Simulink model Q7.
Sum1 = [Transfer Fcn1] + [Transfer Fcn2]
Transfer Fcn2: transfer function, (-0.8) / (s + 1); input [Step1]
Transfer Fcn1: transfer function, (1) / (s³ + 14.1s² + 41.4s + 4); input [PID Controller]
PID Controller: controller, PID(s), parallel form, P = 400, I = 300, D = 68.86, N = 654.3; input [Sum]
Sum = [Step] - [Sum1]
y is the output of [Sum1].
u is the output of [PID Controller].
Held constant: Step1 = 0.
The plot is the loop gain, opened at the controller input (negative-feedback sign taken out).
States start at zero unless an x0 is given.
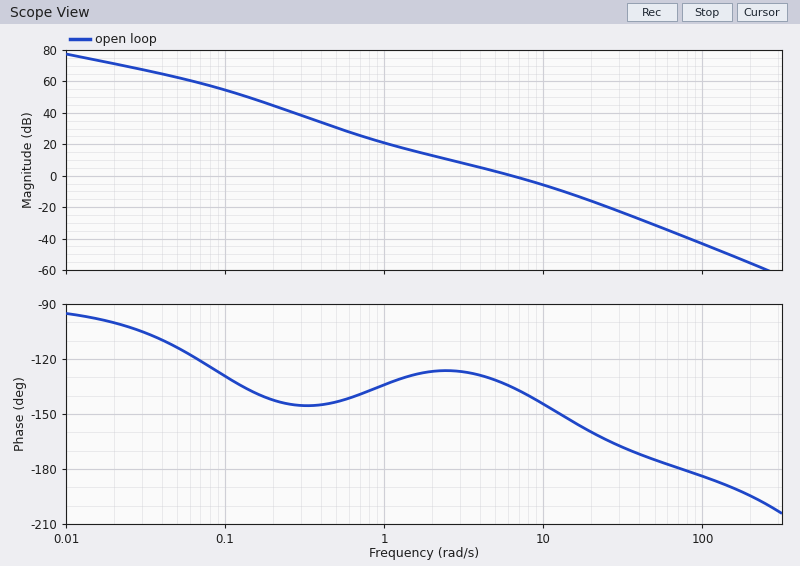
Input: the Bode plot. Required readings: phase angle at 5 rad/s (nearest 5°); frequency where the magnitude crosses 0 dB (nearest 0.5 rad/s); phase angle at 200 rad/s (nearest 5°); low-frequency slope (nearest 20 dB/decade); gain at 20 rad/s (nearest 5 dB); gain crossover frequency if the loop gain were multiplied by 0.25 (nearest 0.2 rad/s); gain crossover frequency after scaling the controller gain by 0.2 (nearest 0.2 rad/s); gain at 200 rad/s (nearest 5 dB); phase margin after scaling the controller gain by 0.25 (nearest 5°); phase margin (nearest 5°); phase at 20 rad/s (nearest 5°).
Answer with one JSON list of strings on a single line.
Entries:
["-130°", "6.5 rad/s", "-195°", "-20 dB/decade", "-15 dB", "2.2 rad/s", "1.8 rad/s", "-55 dB", "55°", "45°", "-160°"]
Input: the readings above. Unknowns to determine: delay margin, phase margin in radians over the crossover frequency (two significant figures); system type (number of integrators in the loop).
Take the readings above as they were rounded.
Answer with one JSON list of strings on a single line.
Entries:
["0.12 s", "1"]
